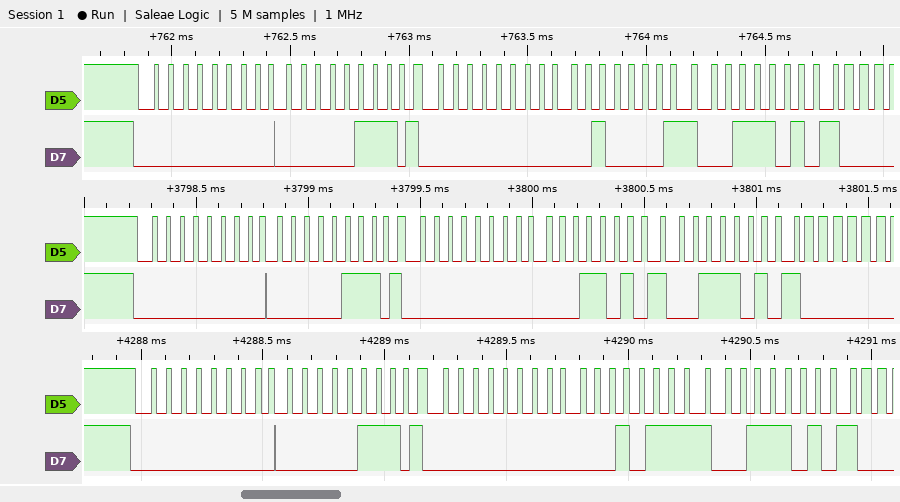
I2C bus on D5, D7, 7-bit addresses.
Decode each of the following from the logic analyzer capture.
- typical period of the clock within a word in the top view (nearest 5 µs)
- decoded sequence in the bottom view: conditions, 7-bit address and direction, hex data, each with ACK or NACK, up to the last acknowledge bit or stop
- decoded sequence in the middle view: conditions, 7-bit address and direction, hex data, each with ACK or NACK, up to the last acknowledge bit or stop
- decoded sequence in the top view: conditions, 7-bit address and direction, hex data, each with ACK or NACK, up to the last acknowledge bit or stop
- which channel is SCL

60 µs
start, address 00 write ACK, 07 ACK, repeated start, address 00 write ACK, 17 NACK, 3A NACK
start, address 00 write ACK, 07 ACK, repeated start, address 00 write ACK, 1A NACK, 3A NACK
start, address 00 write ACK, 07 ACK, repeated start, address 00 write ACK, 21 NACK, 3A NACK
D5
